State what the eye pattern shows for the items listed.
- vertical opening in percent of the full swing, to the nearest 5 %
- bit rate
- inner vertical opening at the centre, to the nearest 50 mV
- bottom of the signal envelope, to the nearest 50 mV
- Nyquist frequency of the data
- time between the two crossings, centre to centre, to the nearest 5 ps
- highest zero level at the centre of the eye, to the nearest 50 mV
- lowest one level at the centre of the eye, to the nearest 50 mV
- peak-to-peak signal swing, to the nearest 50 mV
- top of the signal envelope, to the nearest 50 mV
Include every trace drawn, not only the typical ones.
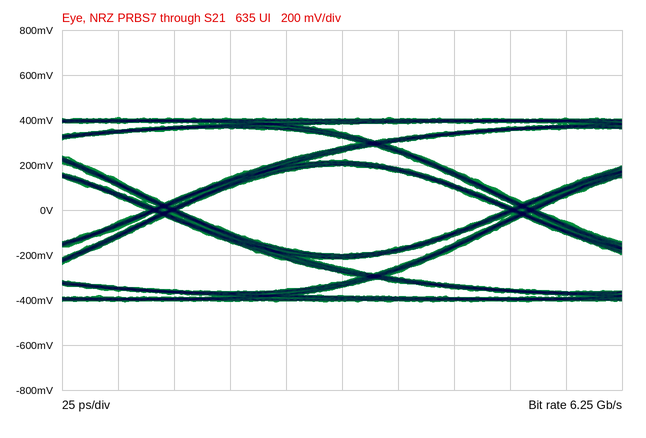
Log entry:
50 %
6.25 Gb/s
400 mV
-400 mV
3.125 GHz
160 ps
-200 mV
200 mV
800 mV
400 mV
